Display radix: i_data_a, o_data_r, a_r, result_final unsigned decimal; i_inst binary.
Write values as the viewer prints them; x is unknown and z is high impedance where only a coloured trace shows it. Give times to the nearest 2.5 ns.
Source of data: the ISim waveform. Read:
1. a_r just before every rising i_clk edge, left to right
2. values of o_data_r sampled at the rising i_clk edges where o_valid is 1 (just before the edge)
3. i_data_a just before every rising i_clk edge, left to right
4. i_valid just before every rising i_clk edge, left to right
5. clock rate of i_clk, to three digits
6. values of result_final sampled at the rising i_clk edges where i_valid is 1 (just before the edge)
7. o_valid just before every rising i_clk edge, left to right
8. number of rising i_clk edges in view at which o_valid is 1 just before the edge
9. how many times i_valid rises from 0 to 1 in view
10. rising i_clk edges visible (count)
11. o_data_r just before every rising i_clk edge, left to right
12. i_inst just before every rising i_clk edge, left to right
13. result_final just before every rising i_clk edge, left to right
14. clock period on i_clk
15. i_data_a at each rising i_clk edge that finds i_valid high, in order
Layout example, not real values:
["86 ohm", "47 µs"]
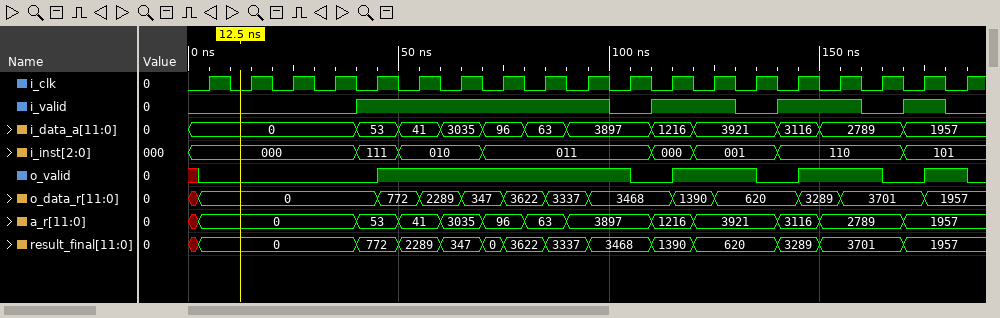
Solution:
["0, 0, 0, 0, 53, 41, 3035, 96, 63, 3897, 3897, 1216, 3921, 3921, 3116, 2789, 2789, 1957, 1957", "772, 2289, 347, 3622, 3337, 3468, 1390, 620, 3289, 3701, 1957", "0, 0, 0, 0, 53, 41, 3035, 96, 63, 3897, 3897, 1216, 3921, 3921, 3116, 2789, 2789, 1957, 1957", "0 0 0 0 1 1 1 1 1 1 0 1 1 0 1 1 0 1 0", "100 MHz", "772, 2289, 347, 0, 3622, 3337, 1390, 620, 3289, 3701, 1957", "0 0 0 0 0 1 1 1 1 1 1 0 1 1 0 1 1 0 1", "11", "4", "19", "0, 0, 0, 0, 0, 772, 2289, 347, 3622, 3337, 3468, 3468, 1390, 620, 620, 3289, 3701, 3701, 1957", "000, 000, 000, 000, 111, 010, 010, 011, 011, 011, 011, 000, 001, 001, 110, 110, 110, 101, 101", "0, 0, 0, 0, 772, 2289, 347, 0, 3622, 3337, 3468, 1390, 620, 620, 3289, 3701, 3701, 1957, 1957", "10 ns", "53, 41, 3035, 96, 63, 3897, 1216, 3921, 3116, 2789, 1957"]
